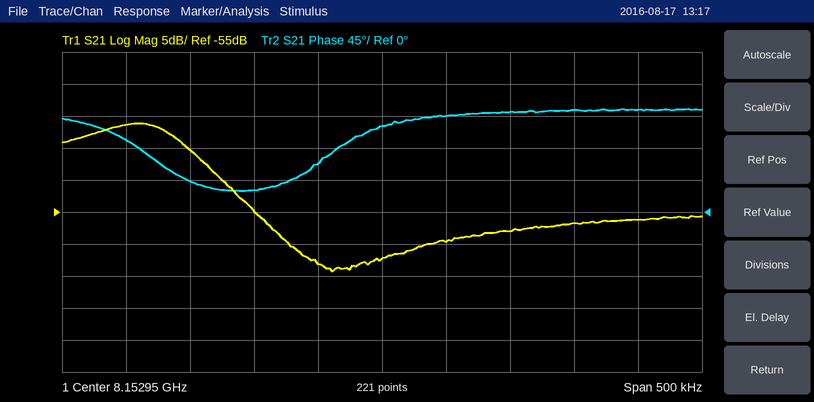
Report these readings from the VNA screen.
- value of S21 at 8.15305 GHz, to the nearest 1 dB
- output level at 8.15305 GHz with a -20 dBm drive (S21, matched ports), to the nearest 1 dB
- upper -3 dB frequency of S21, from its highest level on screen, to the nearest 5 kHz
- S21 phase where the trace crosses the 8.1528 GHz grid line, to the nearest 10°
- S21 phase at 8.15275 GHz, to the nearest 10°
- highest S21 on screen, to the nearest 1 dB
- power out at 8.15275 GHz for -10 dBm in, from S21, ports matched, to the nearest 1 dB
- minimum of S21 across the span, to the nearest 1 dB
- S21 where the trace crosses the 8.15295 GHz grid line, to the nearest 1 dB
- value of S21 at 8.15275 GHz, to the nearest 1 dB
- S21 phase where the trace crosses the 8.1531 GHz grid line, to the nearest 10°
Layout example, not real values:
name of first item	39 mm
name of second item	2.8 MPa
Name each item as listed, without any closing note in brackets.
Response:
value of S21 at 8.15305 GHz, to the nearest 1 dB	-58 dB
output level at 8.15305 GHz with a -20 dBm drive (S21, matched ports), to the nearest 1 dB	-78 dBm
upper -3 dB frequency of S21, from its highest level on screen, to the nearest 5 kHz	8.152795 GHz
S21 phase where the trace crosses the 8.1528 GHz grid line, to the nearest 10°	40°
S21 phase at 8.15275 GHz, to the nearest 10°	100°
highest S21 on screen, to the nearest 1 dB	-41 dB
power out at 8.15275 GHz for -10 dBm in, from S21, ports matched, to the nearest 1 dB	-51 dBm
minimum of S21 across the span, to the nearest 1 dB	-64 dB
S21 where the trace crosses the 8.15295 GHz grid line, to the nearest 1 dB	-62 dB
value of S21 at 8.15275 GHz, to the nearest 1 dB	-41 dB
S21 phase where the trace crosses the 8.1531 GHz grid line, to the nearest 10°	140°
